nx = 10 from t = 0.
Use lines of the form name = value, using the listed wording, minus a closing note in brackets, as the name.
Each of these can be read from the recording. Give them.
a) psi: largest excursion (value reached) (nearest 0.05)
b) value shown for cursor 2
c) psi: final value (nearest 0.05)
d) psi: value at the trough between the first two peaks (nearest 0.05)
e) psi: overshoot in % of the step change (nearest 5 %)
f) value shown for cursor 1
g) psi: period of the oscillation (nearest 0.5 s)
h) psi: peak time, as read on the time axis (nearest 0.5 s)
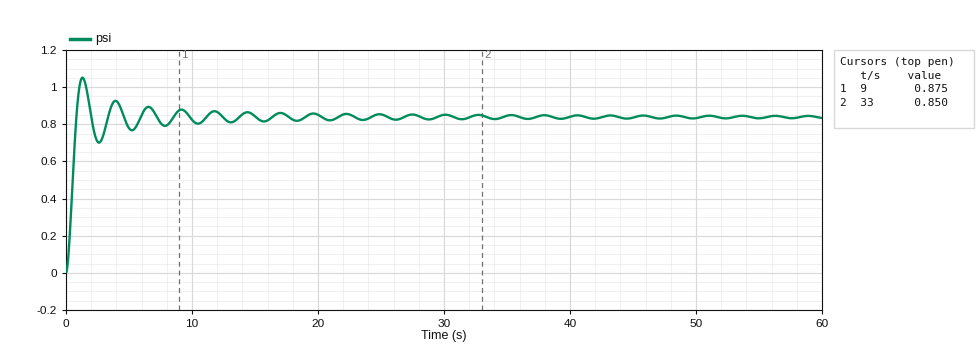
psi: largest excursion (value reached) = 1.05
value shown for cursor 2 = 0.850
psi: final value = 0.85
psi: value at the trough between the first two peaks = 0.70
psi: overshoot in % of the step change = 25 %
value shown for cursor 1 = 0.875
psi: period of the oscillation = 2.5 s
psi: peak time, as read on the time axis = 1.5 s
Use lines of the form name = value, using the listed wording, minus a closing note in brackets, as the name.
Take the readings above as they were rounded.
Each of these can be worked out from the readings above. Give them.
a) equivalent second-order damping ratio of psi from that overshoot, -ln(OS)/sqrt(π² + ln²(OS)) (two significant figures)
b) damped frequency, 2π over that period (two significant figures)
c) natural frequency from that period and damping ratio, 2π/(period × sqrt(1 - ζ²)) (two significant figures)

equivalent second-order damping ratio of psi from that overshoot, -ln(OS)/sqrt(π² + ln²(OS)) = 0.40
damped frequency, 2π over that period = 2.5 rad/s
natural frequency from that period and damping ratio, 2π/(period × sqrt(1 - ζ²)) = 2.7 rad/s
